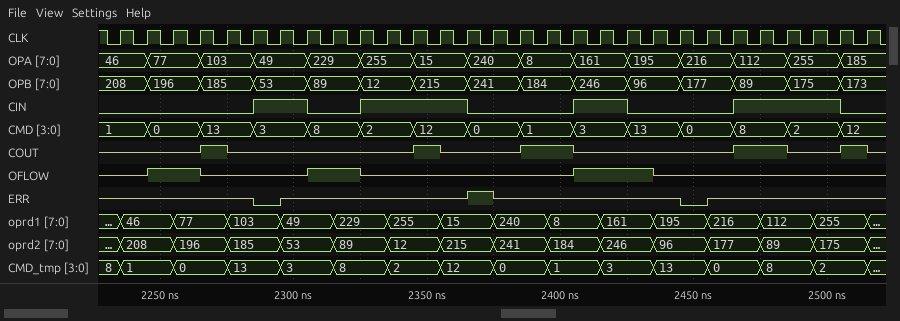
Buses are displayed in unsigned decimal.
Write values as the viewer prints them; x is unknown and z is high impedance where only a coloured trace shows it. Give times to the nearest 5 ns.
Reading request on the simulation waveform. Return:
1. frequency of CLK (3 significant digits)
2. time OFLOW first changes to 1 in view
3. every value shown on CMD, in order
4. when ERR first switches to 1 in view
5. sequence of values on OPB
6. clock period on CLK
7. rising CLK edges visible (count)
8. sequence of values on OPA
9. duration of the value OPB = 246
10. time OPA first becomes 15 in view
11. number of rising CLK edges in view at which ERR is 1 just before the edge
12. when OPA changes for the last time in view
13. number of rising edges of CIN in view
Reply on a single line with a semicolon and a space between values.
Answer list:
100 MHz; 2245 ns; 1, 0, 13, 3, 8, 2, 12, 0, 1, 3, 13, 0, 8, 2, 12; 2365 ns; 208, 196, 185, 53, 89, 12, 215, 241, 184, 246, 96, 177, 89, 175, 173; 10 ns; 29; 46, 77, 103, 49, 229, 255, 15, 240, 8, 161, 195, 216, 112, 255, 185; 20 ns; 2345 ns; 1; 2505 ns; 4
